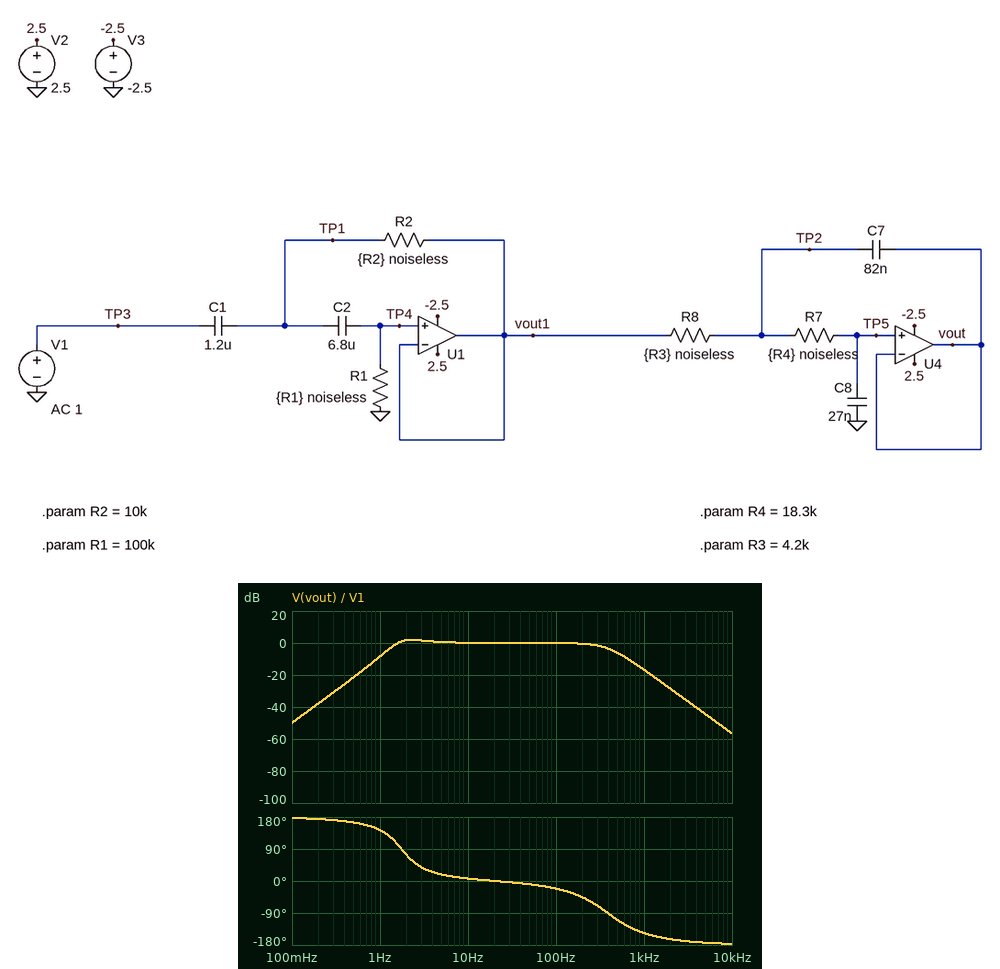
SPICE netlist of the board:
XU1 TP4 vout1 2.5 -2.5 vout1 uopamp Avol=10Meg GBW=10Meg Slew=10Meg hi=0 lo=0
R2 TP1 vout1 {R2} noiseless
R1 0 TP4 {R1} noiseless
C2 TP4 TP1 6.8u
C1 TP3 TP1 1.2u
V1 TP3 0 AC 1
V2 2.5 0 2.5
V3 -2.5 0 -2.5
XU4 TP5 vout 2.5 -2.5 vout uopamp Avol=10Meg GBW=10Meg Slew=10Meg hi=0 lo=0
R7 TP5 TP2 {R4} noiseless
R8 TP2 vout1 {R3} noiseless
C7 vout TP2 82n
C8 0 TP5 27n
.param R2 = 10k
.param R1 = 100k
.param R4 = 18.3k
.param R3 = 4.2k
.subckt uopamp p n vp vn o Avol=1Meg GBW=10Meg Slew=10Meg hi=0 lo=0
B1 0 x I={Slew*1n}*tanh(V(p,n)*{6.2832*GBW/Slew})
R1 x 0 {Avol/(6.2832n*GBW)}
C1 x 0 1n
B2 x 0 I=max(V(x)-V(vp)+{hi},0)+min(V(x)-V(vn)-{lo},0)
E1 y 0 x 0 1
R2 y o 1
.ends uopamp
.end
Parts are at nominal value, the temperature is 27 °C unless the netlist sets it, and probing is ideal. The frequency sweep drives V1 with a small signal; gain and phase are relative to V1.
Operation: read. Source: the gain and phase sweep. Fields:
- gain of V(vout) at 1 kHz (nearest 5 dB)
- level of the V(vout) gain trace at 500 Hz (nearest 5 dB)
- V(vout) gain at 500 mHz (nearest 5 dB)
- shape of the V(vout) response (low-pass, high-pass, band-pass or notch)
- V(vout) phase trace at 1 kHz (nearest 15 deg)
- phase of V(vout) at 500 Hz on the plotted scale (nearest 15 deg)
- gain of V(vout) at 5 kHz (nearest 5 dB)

-15 dB
-5 dB
-20 dB
band-pass
-150 deg
-105 deg
-45 dB
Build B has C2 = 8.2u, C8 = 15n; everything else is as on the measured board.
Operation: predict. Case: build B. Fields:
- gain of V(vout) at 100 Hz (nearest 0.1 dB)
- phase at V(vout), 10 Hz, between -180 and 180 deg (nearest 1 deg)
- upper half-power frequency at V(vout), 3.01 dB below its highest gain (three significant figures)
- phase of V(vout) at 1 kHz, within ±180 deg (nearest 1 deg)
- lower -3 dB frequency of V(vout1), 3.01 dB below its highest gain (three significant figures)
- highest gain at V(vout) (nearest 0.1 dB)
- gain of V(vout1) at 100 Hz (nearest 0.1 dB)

0.1 dB
8 deg
553 Hz
-142 deg
1.36 Hz
1.6 dB
0 dB
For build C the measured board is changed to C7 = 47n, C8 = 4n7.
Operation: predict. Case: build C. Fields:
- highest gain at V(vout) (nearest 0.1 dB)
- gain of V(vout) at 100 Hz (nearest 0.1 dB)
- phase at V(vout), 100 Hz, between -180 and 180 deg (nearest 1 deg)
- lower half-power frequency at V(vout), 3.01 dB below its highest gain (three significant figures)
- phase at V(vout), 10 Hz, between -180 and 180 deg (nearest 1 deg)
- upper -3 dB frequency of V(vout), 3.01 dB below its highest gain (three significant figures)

2.6 dB
0 dB
-3 deg
1.55 Hz
9 deg
1.45 kHz
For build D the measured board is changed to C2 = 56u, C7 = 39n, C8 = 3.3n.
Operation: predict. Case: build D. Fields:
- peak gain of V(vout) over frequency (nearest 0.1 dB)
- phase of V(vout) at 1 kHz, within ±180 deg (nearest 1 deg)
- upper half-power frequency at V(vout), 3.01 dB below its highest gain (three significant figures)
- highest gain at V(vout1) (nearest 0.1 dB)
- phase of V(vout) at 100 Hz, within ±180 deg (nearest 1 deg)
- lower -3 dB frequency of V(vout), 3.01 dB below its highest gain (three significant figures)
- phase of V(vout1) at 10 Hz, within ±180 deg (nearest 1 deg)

3.2 dB
-37 deg
1.90 kHz
0 dB
-2 deg
272 Hz
8 deg
